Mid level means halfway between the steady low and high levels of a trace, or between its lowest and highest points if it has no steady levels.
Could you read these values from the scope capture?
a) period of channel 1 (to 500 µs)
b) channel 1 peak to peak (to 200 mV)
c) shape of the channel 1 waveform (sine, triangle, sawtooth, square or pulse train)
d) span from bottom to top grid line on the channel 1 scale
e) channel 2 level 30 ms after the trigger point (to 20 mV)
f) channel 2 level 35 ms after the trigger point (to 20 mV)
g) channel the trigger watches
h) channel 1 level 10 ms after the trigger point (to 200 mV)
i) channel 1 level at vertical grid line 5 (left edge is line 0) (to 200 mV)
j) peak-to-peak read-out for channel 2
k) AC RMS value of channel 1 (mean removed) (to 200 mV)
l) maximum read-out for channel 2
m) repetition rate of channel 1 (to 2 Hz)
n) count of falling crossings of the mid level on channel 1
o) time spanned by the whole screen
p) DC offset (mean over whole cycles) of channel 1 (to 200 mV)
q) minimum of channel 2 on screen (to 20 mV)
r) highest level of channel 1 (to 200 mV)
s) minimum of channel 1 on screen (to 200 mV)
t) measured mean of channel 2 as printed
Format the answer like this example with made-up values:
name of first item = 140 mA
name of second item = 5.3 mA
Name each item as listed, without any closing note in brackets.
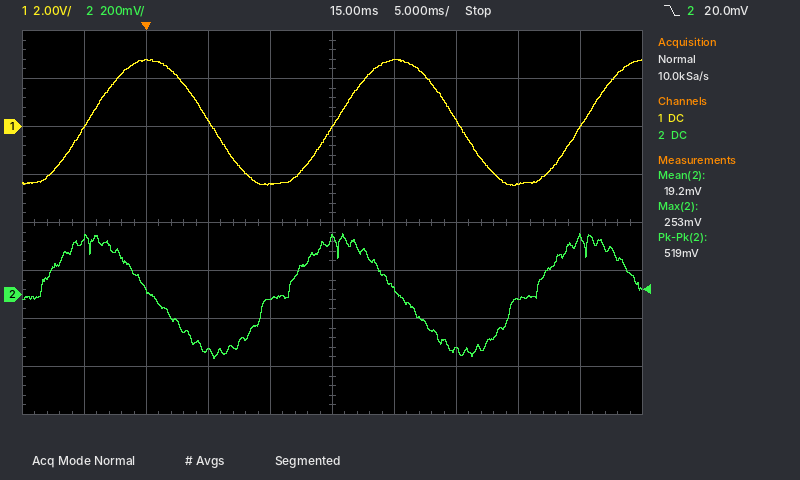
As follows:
period of channel 1 = 20.0 ms
channel 1 peak to peak = 5.2 V
shape of the channel 1 waveform = sine
span from bottom to top grid line on the channel 1 scale = 16 V
channel 2 level 30 ms after the trigger point = -20 mV
channel 2 level 35 ms after the trigger point = 240 mV
channel the trigger watches = channel 2
channel 1 level 10 ms after the trigger point = -2.4 V
channel 1 level at vertical grid line 5 (left edge is line 0) = 0.0 V
peak-to-peak read-out for channel 2 = 519 mV
AC RMS value of channel 1 (mean removed) = 1.8 V
maximum read-out for channel 2 = 253 mV
repetition rate of channel 1 = 50 Hz
count of falling crossings of the mid level on channel 1 = 2
time spanned by the whole screen = 50 ms
DC offset (mean over whole cycles) of channel 1 = 200 mV
minimum of channel 2 on screen = -260 mV
highest level of channel 1 = 2.8 V
minimum of channel 1 on screen = -2.4 V
measured mean of channel 2 as printed = 19.2 mV
